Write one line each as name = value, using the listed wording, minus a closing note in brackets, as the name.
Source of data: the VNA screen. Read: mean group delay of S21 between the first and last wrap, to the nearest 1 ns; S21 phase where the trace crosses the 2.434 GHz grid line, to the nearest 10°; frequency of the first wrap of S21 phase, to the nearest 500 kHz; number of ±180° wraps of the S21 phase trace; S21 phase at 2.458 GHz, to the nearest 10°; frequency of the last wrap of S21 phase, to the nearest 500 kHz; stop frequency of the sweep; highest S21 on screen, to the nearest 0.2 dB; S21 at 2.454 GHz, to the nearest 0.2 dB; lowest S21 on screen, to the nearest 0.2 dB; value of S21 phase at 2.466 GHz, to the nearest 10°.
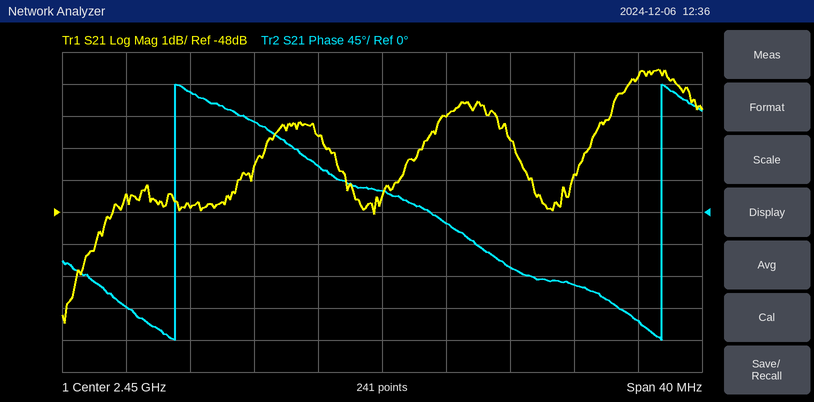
mean group delay of S21 between the first and last wrap, to the nearest 1 ns = 33 ns
S21 phase where the trace crosses the 2.434 GHz grid line, to the nearest 10° = -130°
frequency of the first wrap of S21 phase, to the nearest 500 kHz = 2.4370 GHz
number of ±180° wraps of the S21 phase trace = 2
S21 phase at 2.458 GHz, to the nearest 10° = -80°
frequency of the last wrap of S21 phase, to the nearest 500 kHz = 2.4675 GHz
stop frequency of the sweep = 2.47 GHz
highest S21 on screen, to the nearest 0.2 dB = -43.6 dB
S21 at 2.454 GHz, to the nearest 0.2 dB = -45.0 dB
lowest S21 on screen, to the nearest 0.2 dB = -51.4 dB
value of S21 phase at 2.466 GHz, to the nearest 10° = -150°
